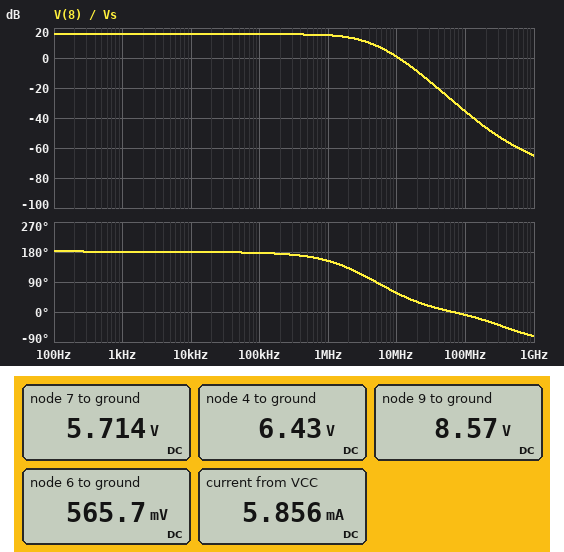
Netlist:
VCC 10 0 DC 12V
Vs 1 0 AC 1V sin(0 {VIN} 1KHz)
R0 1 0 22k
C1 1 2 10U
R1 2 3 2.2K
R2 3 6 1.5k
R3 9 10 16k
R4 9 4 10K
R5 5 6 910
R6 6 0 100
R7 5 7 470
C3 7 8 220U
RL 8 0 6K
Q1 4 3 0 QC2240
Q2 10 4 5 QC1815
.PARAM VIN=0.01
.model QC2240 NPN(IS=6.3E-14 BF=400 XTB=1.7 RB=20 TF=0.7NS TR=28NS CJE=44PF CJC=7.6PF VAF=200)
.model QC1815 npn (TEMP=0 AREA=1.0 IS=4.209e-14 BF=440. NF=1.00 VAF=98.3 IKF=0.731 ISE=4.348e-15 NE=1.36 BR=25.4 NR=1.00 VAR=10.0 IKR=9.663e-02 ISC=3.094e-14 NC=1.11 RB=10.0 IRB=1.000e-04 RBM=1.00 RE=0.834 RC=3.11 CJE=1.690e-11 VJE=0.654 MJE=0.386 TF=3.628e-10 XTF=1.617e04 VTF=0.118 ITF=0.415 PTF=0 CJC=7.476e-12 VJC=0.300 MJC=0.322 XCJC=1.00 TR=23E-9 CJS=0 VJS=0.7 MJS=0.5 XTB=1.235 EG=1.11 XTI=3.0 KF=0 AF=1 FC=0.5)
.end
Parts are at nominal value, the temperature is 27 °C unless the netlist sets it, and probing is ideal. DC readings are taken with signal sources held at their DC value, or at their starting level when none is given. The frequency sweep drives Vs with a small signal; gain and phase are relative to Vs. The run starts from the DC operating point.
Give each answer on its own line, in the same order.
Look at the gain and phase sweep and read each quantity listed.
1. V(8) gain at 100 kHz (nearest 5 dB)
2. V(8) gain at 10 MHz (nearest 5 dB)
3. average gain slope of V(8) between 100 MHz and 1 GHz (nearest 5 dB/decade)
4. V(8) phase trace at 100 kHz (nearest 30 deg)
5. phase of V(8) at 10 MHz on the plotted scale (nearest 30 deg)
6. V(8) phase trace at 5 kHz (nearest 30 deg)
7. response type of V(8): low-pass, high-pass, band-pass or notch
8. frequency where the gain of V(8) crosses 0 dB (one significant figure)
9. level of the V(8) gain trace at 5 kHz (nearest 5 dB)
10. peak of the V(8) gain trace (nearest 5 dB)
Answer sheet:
15 dB
0 dB
-30 dB/decade
180 deg
60 deg
180 deg
low-pass
10 MHz
15 dB
15 dB
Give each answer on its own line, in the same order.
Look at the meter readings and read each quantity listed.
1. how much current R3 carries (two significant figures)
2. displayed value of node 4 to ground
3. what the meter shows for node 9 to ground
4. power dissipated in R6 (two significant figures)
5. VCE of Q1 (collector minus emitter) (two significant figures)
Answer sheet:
210 µA
6.43 V
8.57 V
3.2 mW
6.4 V
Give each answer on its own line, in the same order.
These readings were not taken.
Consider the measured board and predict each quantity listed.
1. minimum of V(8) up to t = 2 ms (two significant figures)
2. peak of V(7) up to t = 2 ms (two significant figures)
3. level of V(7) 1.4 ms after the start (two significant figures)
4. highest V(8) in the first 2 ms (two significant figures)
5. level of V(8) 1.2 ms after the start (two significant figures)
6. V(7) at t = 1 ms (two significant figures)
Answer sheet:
-61 mV
5.8 V
5.7 V
62 mV
-58 mV
5.7 V
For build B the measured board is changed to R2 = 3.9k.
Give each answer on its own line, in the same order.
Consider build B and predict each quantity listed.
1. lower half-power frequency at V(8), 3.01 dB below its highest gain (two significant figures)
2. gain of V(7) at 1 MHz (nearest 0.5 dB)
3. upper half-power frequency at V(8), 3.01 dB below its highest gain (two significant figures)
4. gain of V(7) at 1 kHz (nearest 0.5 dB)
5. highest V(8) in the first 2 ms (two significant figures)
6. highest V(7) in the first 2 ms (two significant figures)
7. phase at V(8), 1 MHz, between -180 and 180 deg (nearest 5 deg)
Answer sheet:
6.6 Hz
20.5 dB
1.0 MHz
23.5 dB
150 mV
5.9 V
130 deg
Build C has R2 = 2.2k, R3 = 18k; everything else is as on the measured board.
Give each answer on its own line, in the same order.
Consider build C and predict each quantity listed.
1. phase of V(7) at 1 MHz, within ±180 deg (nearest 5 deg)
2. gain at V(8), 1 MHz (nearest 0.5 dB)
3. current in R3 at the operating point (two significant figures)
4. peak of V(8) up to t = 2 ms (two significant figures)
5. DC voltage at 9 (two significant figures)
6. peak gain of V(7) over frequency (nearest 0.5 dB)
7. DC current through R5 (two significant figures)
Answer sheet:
145 deg
17.5 dB
200 µA
88 mV
8.4 V
19.0 dB
5.6 mA
